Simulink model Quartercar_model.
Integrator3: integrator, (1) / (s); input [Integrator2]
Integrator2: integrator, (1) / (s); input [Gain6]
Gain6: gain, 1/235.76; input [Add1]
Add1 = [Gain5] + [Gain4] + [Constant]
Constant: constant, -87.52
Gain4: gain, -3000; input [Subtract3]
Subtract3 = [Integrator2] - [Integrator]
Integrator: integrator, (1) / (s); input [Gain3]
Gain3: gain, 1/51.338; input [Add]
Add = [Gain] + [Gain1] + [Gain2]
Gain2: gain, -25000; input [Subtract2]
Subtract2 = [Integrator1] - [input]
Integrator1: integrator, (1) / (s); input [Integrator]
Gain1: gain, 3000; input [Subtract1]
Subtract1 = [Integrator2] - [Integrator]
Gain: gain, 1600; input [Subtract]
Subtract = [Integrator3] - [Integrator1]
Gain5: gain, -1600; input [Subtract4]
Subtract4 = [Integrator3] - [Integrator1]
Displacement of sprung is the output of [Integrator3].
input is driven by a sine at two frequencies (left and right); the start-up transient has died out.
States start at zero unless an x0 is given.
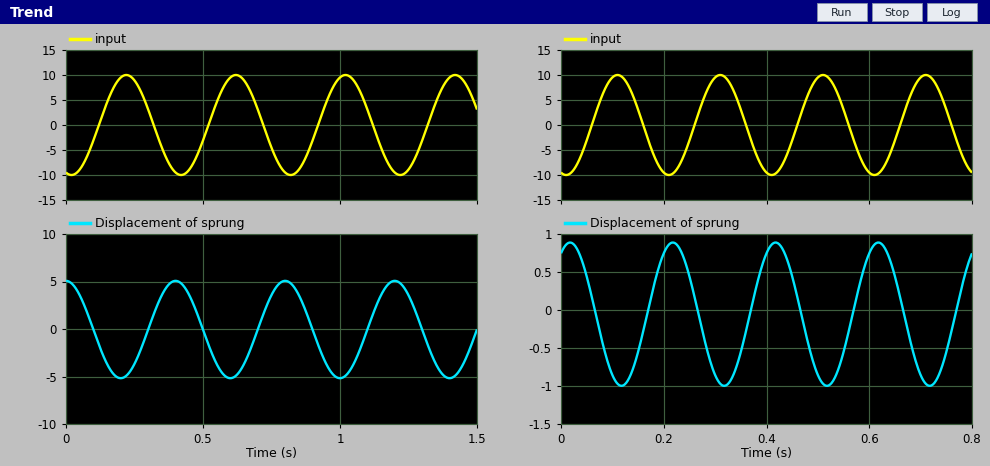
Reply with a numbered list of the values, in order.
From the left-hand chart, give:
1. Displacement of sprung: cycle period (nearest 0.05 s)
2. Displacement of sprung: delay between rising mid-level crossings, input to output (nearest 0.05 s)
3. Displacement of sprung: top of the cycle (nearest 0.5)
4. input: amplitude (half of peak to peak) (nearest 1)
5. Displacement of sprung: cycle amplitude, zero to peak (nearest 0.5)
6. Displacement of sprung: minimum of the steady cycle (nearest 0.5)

1. 0.40 s
2. 0.20 s
3. 5.0
4. 10
5. 5.0
6. -5.0
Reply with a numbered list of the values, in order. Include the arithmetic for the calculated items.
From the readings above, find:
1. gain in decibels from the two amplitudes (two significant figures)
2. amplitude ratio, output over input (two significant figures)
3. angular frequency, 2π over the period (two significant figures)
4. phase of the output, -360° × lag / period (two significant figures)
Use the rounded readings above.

1. 20 log10(5 / 10) = -6.0 dB
2. 5 / 10 = 0.50
3. 2π / 0.4 = 16 rad/s
4. -360 × 0.2 / 0.4 = -180°
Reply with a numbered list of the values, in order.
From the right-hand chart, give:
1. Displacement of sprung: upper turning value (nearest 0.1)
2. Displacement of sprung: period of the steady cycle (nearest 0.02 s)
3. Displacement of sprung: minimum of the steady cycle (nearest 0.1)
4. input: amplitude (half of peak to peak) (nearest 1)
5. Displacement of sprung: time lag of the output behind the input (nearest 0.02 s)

1. 0.9
2. 0.20 s
3. -1.0
4. 10
5. 0.10 s
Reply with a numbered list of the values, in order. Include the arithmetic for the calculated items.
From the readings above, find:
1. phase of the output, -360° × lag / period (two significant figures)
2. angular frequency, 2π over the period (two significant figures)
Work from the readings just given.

1. -360 × 0.1 / 0.2 = -180°
2. 2π / 0.2 = 31 rad/s
